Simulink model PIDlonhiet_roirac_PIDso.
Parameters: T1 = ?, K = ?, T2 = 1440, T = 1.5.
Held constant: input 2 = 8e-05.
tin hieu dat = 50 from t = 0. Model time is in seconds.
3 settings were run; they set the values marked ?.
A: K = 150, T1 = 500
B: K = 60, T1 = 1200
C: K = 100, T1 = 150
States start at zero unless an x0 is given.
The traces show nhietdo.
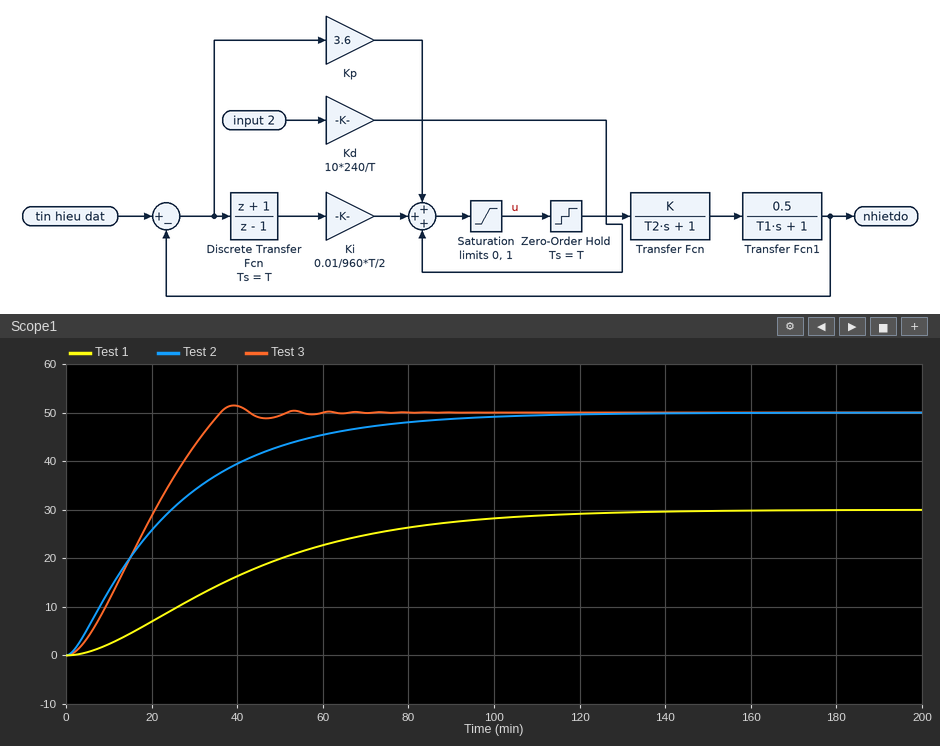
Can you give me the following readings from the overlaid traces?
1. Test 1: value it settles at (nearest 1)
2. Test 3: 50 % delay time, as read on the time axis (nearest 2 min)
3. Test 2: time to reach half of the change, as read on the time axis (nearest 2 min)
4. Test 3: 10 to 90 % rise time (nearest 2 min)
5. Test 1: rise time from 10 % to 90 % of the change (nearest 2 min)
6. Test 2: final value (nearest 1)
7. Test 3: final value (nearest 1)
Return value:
30
18 min
20 min
26 min
74 min
50
50
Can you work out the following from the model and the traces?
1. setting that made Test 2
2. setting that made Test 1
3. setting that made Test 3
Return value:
C
B
A
